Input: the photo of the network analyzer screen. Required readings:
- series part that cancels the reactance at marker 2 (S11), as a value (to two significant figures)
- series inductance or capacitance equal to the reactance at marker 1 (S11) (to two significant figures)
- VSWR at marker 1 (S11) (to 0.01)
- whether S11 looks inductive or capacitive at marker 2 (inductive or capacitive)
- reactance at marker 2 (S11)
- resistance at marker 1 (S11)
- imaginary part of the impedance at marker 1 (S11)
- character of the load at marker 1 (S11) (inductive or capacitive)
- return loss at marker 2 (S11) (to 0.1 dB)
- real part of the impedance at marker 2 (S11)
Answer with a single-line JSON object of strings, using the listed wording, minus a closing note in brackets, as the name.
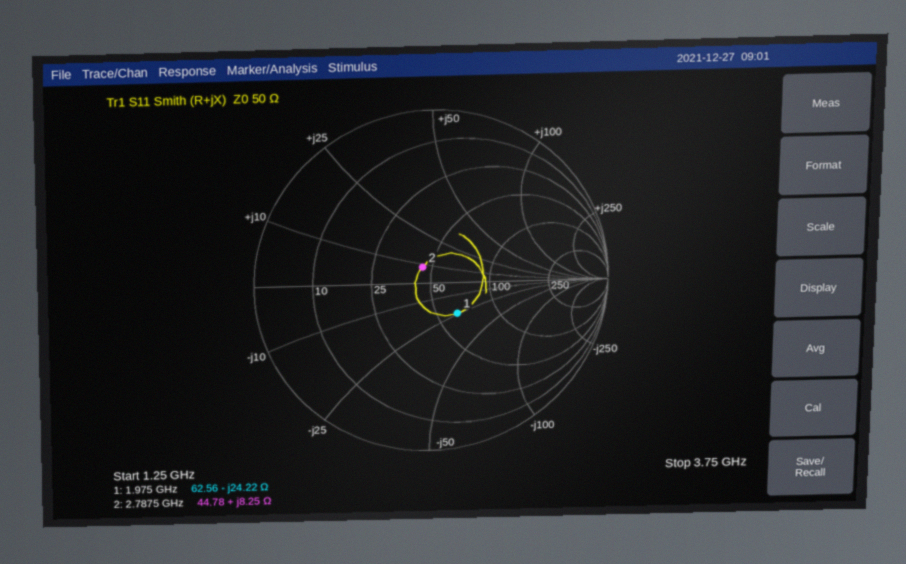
{"series part that cancels the reactance at marker 2 (S11), as a value": "6.9 pF", "series inductance or capacitance equal to the reactance at marker 1 (S11)": "3.3 pF", "VSWR at marker 1 (S11)": "1.62", "whether S11 looks inductive or capacitive at marker 2": "inductive", "reactance at marker 2": "+8.25 Ω", "resistance at marker 1": "62.56 Ω", "imaginary part of the impedance at marker 1": "-24.22 Ω", "character of the load at marker 1 (S11)": "capacitive", "return loss at marker 2 (S11)": "19.8 dB", "real part of the impedance at marker 2": "44.78 Ω"}
